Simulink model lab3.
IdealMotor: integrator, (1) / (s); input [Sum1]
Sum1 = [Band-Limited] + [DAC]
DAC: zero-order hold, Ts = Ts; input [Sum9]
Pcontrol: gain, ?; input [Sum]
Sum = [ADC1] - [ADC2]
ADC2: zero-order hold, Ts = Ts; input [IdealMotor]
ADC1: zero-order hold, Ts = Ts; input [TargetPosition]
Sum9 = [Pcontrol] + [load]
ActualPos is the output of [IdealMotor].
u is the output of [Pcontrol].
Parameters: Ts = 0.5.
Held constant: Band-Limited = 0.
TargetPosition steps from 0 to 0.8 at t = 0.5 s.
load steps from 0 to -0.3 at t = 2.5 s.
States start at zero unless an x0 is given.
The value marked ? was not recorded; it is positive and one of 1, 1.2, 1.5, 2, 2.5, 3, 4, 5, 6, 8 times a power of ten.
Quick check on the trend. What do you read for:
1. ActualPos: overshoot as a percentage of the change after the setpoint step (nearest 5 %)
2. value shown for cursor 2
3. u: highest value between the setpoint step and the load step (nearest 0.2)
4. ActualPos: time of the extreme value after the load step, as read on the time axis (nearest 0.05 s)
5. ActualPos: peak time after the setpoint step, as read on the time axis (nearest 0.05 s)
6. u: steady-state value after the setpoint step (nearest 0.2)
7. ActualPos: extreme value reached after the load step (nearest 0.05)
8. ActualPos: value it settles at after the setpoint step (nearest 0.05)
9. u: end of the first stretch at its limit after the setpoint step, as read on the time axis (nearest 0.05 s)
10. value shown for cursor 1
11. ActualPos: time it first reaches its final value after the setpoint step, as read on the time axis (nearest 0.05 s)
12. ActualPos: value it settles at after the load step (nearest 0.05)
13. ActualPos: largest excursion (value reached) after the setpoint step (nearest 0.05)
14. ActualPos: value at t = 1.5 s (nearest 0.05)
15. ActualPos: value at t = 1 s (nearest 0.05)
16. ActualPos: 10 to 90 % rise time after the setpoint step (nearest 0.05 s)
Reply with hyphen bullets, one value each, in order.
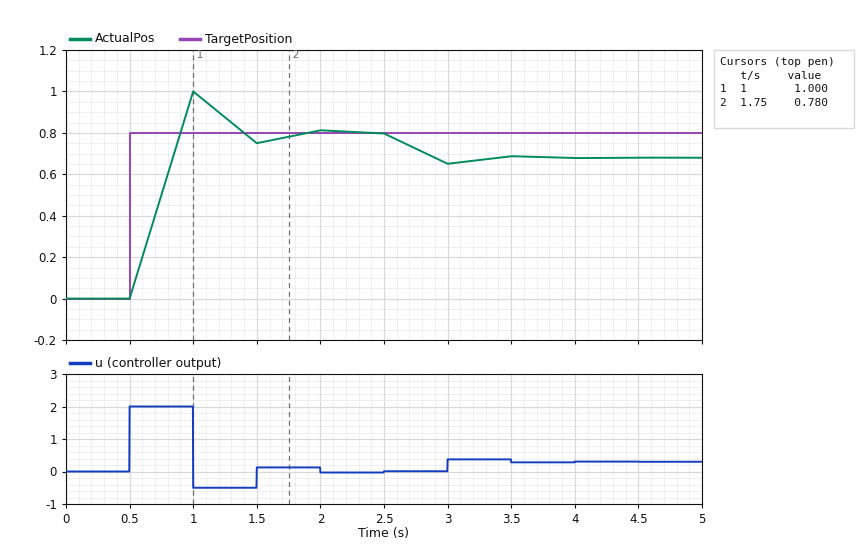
- 25 %
- 0.780
- 2.0
- 3.00 s
- 1.00 s
- 0.0
- 0.65
- 0.80
- 1.00 s
- 1.000
- 0.90 s
- 0.70
- 1.00
- 0.75
- 1.00
- 0.30 s
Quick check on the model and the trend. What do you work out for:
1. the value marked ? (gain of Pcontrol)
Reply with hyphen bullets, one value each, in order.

- 2.5
